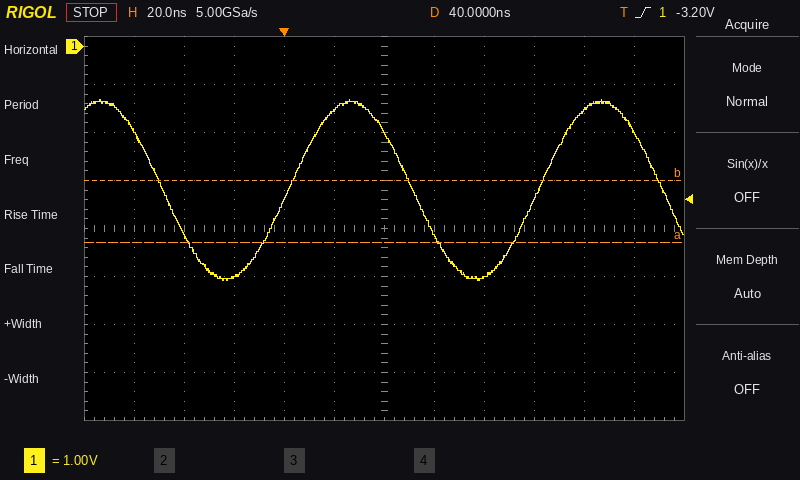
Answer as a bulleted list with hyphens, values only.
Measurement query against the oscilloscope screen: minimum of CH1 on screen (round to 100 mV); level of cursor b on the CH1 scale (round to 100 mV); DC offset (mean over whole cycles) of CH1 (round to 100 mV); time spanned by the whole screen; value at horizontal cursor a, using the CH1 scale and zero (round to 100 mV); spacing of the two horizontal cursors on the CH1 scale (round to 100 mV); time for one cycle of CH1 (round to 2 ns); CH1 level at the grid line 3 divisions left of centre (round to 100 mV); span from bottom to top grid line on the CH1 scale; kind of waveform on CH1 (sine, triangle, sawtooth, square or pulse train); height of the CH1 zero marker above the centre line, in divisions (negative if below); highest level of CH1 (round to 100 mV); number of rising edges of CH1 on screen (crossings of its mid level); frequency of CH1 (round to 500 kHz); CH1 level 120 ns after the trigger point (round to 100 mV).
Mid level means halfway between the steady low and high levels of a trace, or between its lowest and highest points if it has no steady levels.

- -4.9 V
- -2.8 V
- -3.0 V
- 240 ns
- -4.1 V
- 1.3 V
- 100 ns
- -4.8 V
- 8 V
- sine
- +3.8 div
- -1.1 V
- 2
- 10.0 MHz
- -1.3 V
